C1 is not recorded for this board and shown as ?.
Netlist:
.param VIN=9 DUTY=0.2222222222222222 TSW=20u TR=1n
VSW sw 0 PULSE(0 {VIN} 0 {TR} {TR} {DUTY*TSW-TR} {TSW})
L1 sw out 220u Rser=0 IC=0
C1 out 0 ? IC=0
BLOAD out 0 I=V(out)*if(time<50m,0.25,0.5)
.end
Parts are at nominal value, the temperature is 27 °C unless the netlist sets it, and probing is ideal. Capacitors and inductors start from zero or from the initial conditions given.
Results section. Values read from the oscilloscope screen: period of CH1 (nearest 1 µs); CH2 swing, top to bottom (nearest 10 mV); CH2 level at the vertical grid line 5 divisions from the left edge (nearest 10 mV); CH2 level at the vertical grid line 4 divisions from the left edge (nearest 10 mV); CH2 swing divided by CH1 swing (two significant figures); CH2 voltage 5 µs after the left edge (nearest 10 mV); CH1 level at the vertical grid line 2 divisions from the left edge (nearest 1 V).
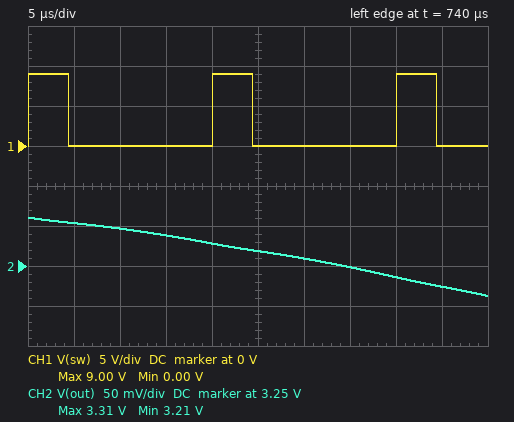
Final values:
20 µs
100 mV
3.27 V
3.28 V
0.011
3.30 V
0 V
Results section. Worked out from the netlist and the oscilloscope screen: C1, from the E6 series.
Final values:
220 µF
